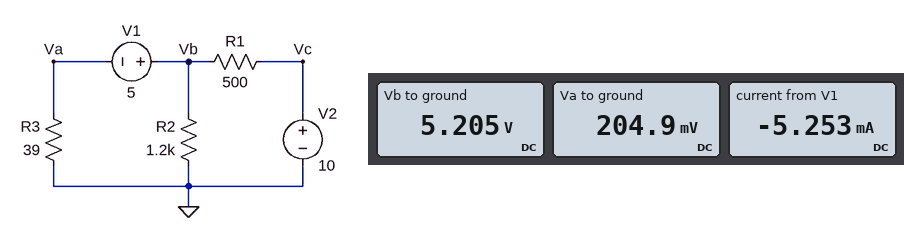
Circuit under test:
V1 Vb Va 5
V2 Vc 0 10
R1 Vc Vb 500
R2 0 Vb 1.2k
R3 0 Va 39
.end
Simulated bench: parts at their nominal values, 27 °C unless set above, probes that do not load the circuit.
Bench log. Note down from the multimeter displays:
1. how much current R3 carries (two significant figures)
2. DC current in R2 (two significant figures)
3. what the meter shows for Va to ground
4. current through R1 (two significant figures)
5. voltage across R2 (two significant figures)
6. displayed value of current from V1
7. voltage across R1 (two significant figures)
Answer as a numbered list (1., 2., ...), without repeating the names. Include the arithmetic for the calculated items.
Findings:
1. (204.9 mV) / 39 Ω = 5.3 mA
2. (5.205 V) / 1.2 kΩ = 4.3 mA
3. 204.9 mV
4. (10 V - 5.205 V) / 500 Ω = 9.6 mA
5. 5.205 V = 5.2 V
6. -5.253 mA
7. 10 V - 5.205 V = 4.8 V
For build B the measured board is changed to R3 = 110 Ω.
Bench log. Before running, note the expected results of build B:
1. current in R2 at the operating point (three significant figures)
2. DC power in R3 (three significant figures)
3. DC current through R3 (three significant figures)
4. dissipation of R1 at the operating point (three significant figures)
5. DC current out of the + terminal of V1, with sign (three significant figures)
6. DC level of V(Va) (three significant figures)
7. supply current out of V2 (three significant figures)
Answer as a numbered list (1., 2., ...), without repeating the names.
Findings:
1. 4.57 mA
2. 2.18 mW
3. 4.45 mA
4. 40.7 mW
5. -4.45 mA
6. 489 mV
7. 9.02 mA
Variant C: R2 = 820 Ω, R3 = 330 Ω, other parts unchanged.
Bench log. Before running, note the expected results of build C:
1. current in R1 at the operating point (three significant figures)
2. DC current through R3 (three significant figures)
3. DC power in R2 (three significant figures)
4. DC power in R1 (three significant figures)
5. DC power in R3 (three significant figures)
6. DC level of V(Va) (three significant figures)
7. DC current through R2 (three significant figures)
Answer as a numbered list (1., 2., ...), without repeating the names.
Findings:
1. 8.75 mA
2. 1.89 mA
3. 38.6 mW
4. 38.3 mW
5. 1.18 mW
6. 624 mV
7. 6.86 mA
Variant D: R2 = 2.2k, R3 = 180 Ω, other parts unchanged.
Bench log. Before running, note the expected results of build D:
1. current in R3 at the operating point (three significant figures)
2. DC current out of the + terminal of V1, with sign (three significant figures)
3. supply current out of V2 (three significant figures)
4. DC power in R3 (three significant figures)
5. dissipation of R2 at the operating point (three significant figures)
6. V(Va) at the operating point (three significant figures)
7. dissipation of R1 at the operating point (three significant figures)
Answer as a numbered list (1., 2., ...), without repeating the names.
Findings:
1. 5.36 mA
2. -5.36 mA
3. 8.07 mA
4. 5.17 mW
5. 16.2 mW
6. 965 mV
7. 32.6 mW
